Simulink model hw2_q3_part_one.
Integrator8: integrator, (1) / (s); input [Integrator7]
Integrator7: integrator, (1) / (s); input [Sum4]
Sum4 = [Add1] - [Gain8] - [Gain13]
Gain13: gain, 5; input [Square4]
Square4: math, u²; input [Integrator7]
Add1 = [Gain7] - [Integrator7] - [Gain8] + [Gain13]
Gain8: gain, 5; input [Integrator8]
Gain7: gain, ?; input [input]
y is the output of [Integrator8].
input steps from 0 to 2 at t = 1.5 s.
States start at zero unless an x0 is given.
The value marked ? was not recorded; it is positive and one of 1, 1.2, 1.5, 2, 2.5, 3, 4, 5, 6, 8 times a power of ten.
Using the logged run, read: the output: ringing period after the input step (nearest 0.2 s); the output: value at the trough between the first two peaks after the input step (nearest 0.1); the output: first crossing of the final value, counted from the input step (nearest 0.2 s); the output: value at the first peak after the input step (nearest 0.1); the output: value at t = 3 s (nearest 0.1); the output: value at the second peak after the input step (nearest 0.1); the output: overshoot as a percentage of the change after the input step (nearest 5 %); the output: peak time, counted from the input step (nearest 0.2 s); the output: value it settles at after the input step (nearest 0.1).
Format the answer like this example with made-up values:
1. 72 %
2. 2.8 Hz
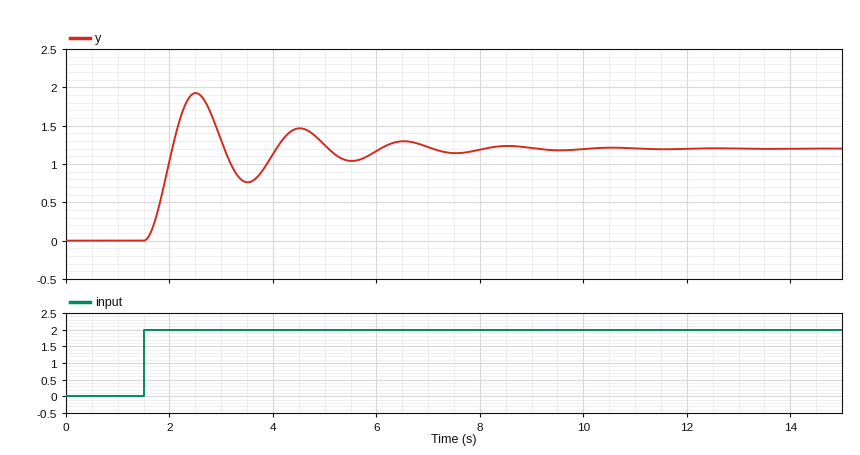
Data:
1. 2.0 s
2. 0.8
3. 0.6 s
4. 1.9
5. 1.3
6. 1.5
7. 60 %
8. 1.0 s
9. 1.2
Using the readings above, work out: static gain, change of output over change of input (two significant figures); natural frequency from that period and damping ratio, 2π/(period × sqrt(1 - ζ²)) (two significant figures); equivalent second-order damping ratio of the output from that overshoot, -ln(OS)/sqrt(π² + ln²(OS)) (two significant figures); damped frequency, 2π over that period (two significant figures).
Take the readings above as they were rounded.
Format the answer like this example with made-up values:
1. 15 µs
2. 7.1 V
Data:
1. 0.60
2. 3.2 rad/s
3. 0.16
4. 3.1 rad/s
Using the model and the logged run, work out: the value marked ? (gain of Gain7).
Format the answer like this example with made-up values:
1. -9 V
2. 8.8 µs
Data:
1. 6
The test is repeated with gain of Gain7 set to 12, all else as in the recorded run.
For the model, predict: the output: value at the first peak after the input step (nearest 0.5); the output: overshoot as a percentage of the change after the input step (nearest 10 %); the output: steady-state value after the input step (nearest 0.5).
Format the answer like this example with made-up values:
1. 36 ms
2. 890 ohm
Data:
1. 4.0
2. 60 %
3. 2.5
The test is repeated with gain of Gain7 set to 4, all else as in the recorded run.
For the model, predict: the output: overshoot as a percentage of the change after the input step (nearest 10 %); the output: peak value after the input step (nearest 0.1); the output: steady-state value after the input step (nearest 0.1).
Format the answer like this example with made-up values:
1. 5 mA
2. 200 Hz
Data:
1. 60 %
2. 1.3
3. 0.8
